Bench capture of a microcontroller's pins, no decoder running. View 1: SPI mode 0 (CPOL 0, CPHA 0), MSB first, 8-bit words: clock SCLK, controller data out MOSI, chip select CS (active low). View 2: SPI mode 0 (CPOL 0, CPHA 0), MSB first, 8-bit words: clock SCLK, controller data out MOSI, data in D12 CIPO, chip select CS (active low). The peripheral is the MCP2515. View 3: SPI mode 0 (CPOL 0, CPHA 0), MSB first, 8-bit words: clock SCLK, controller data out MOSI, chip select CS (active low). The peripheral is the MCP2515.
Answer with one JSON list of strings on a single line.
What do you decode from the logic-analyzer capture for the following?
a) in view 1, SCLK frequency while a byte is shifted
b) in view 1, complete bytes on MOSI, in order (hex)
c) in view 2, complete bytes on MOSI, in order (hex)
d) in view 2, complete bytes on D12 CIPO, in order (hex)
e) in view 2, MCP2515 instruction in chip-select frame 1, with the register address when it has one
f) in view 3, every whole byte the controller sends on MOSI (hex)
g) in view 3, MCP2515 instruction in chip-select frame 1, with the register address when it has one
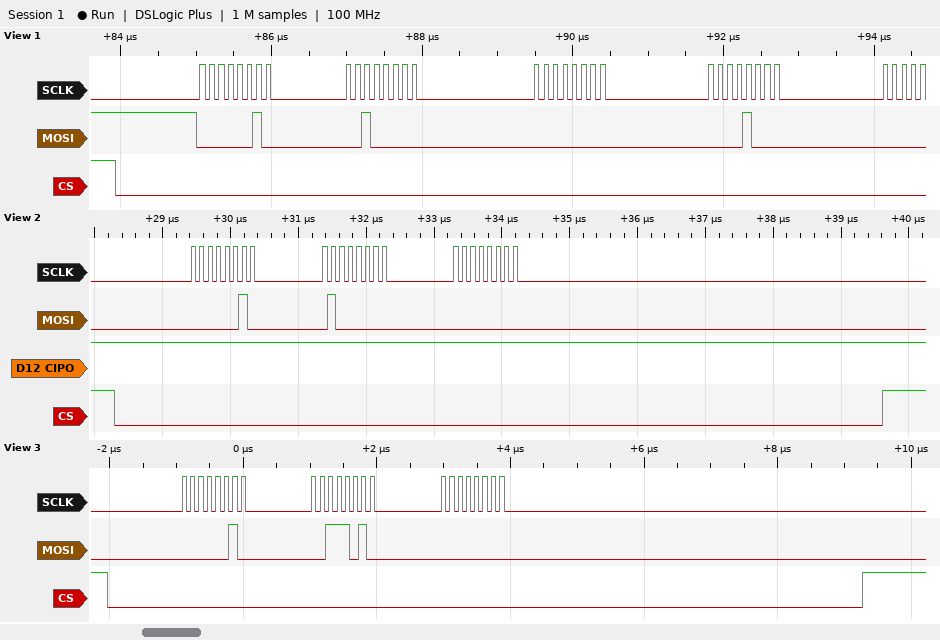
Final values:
["8 MHz", "02 20 00 08", "02 40 00", "FF FF FF", "WRITE 0x40", "02 3A 00", "WRITE 0x3A"]
